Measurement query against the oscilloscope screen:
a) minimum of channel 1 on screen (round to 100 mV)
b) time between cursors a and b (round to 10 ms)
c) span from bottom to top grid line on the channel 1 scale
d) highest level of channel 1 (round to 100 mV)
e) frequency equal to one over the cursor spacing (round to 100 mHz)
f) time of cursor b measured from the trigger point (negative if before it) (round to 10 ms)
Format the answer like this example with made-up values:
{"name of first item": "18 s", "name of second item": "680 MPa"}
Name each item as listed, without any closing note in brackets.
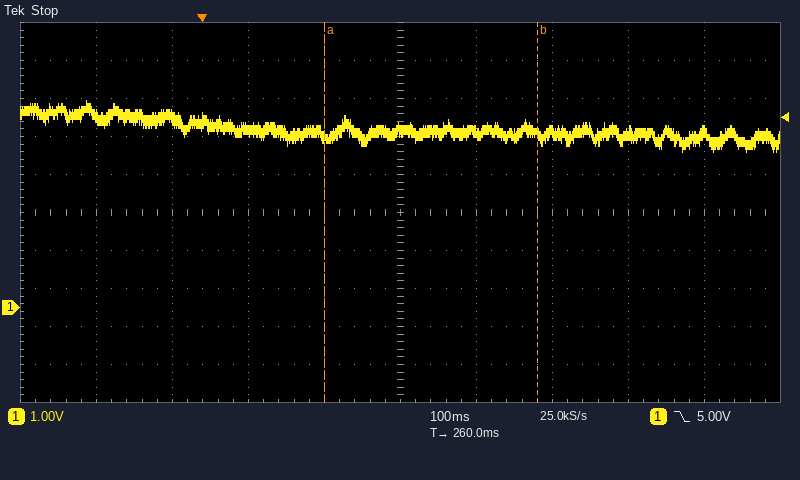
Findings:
{"minimum of channel 1 on screen": "4.1 V", "time between cursors a and b": "280 ms", "span from bottom to top grid line on the channel 1 scale": "10 V", "highest level of channel 1": "5.4 V", "frequency equal to one over the cursor spacing": "3.6 Hz", "time of cursor b measured from the trigger point (negative if before it)": "+440 ms"}
